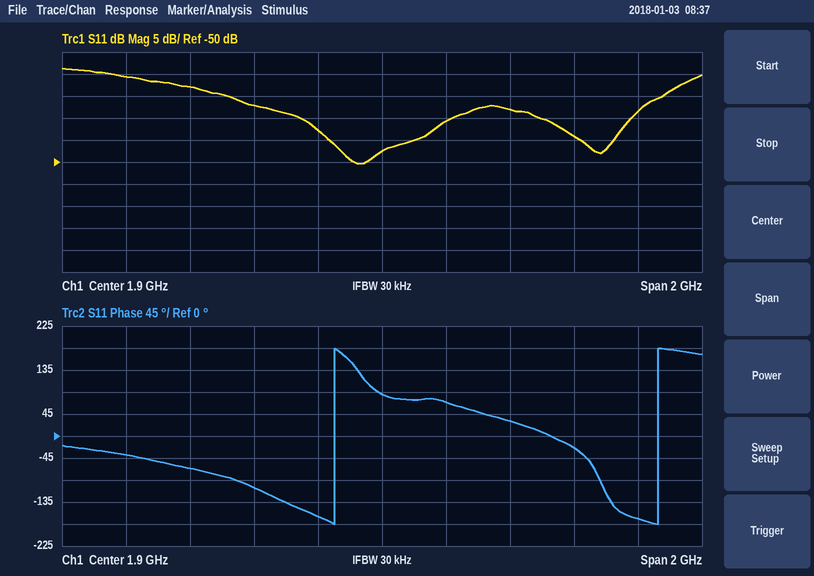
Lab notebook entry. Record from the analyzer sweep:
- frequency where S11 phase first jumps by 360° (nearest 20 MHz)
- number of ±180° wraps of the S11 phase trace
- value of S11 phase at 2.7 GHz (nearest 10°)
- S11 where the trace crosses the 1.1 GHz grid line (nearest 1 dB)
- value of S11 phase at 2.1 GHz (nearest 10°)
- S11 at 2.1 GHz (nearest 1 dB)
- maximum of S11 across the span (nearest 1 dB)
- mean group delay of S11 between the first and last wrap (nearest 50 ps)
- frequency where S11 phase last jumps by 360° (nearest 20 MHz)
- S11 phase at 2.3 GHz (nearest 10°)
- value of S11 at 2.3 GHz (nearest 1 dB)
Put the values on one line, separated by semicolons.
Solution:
1.76 GHz; 2; -170°; -31 dB; 70°; -41 dB; -29 dB; 1.00 ns; 2.76 GHz; 30°; -38 dB
